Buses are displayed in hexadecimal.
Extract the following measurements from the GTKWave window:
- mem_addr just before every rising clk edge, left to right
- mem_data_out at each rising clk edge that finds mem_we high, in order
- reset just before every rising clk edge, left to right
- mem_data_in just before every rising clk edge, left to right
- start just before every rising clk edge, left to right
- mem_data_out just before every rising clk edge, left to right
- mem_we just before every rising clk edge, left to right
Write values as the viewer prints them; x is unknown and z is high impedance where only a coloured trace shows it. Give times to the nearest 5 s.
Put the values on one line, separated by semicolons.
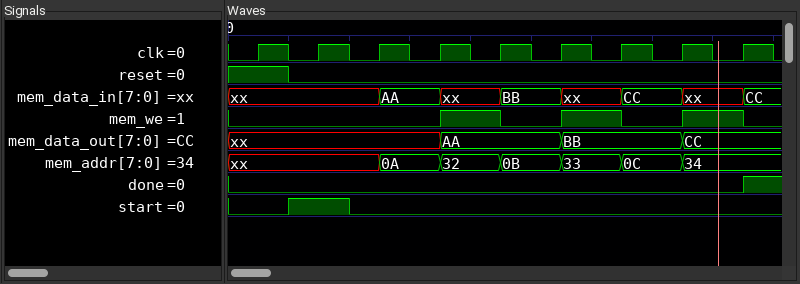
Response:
xx, xx, xx, 0A, 32, 0B, 33, 0C, 34; AA, BB, CC; 1 0 0 0 0 0 0 0 0; xx, xx, xx, AA, xx, BB, xx, CC, xx; 0 1 0 0 0 0 0 0 0; xx, xx, xx, xx, AA, AA, BB, BB, CC; 0 0 0 0 1 0 1 0 1
